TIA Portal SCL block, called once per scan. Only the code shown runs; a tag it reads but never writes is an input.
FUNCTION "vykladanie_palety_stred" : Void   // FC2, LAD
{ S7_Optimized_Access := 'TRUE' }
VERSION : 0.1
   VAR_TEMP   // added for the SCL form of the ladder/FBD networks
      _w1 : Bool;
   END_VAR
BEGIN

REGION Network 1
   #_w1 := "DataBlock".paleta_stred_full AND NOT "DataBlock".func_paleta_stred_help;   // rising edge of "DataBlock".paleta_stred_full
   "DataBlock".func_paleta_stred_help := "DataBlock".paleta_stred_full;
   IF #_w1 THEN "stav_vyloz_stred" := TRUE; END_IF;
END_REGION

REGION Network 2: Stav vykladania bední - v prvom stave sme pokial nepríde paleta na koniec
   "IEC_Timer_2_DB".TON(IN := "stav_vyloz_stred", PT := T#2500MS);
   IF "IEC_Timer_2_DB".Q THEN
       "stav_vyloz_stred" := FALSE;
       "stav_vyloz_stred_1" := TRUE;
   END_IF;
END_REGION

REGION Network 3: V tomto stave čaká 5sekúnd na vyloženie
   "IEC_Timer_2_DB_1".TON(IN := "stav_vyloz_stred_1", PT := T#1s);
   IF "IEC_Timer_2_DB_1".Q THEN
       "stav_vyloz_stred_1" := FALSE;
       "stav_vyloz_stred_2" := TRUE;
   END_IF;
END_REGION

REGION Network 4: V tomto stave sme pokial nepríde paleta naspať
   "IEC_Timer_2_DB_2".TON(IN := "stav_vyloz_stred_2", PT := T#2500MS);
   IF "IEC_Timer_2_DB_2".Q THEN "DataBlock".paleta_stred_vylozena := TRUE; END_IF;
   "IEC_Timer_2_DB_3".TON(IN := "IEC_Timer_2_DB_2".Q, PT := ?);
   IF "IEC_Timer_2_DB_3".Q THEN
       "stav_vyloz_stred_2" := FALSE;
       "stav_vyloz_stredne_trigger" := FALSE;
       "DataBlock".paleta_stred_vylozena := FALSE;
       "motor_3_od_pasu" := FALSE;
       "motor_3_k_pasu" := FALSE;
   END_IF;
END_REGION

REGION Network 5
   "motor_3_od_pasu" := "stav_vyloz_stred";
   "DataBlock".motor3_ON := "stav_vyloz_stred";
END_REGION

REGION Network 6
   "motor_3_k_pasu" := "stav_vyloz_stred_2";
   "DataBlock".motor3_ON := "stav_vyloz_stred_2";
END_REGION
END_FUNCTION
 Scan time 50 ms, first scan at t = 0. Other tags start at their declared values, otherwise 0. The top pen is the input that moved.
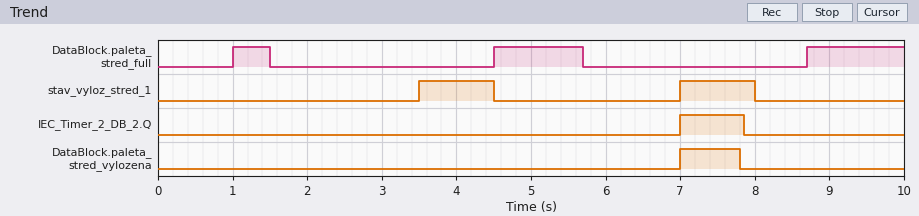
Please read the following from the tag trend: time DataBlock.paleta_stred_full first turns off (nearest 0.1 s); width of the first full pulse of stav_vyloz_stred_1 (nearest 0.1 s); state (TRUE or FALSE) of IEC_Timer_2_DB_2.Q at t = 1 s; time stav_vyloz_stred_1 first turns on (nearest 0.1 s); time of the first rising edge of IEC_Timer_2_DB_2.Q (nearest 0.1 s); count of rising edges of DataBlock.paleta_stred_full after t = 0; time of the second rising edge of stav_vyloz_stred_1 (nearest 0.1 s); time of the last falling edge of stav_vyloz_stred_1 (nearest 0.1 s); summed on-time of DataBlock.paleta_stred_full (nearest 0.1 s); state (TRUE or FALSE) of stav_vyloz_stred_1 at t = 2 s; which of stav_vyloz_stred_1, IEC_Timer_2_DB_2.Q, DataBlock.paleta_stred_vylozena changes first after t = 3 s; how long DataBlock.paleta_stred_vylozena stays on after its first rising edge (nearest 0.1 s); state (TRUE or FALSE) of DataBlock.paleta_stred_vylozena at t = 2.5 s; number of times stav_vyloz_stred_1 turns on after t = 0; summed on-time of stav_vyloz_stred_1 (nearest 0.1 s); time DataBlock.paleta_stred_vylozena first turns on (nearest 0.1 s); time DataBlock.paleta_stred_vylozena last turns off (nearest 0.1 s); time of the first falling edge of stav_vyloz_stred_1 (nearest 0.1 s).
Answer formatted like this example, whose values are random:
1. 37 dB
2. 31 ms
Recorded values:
1. 1.5 s
2. 1.0 s
3. FALSE
4. 3.5 s
5. 7.0 s
6. 3
7. 7.0 s
8. 8.0 s
9. 3.0 s
10. FALSE
11. stav_vyloz_stred_1
12. 0.8 s
13. FALSE
14. 2
15. 2.0 s
16. 7.0 s
17. 7.8 s
18. 4.5 s
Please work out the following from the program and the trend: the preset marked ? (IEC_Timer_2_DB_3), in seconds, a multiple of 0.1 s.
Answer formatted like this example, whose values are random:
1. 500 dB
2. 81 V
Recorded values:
1. 0.8 s
